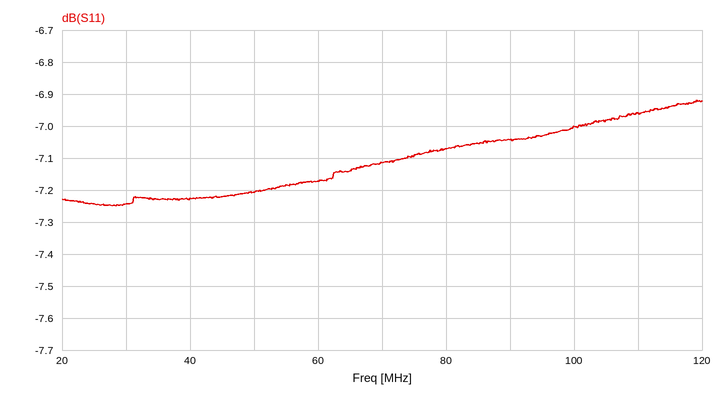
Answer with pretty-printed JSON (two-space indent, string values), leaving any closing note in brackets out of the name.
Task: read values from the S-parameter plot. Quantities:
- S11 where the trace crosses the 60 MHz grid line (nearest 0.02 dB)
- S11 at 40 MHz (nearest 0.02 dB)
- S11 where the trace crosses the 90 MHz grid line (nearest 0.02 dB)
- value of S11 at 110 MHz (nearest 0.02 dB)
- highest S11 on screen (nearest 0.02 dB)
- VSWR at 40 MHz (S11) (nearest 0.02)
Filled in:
{
  "S11 where the trace crosses the 60 MHz grid line": "-7.18 dB",
  "S11 at 40 MHz": "-7.22 dB",
  "S11 where the trace crosses the 90 MHz grid line": "-7.04 dB",
  "value of S11 at 110 MHz": "-6.96 dB",
  "highest S11 on screen": "-6.92 dB",
  "VSWR at 40 MHz (S11)": "2.54"
}
